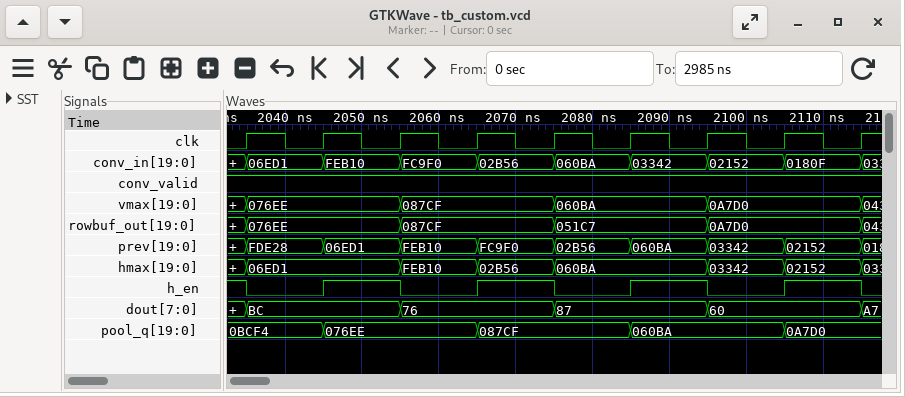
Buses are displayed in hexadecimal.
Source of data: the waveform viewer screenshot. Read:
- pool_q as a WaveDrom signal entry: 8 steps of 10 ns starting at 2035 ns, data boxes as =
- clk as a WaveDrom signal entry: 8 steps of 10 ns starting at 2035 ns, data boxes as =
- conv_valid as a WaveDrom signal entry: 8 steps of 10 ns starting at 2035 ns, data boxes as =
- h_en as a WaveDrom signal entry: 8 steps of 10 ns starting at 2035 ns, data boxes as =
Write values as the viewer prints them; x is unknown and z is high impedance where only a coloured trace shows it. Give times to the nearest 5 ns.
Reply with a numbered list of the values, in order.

1. {name: 'pool_q', wave: '==.=.=.=', data: '0BCF4 076EE 087CF 060BA 0A7D0'}
2. {name: 'clk', wave: 'p.......'}
3. {name: 'conv_valid', wave: '1.......'}
4. {name: 'h_en', wave: '01010101'}
